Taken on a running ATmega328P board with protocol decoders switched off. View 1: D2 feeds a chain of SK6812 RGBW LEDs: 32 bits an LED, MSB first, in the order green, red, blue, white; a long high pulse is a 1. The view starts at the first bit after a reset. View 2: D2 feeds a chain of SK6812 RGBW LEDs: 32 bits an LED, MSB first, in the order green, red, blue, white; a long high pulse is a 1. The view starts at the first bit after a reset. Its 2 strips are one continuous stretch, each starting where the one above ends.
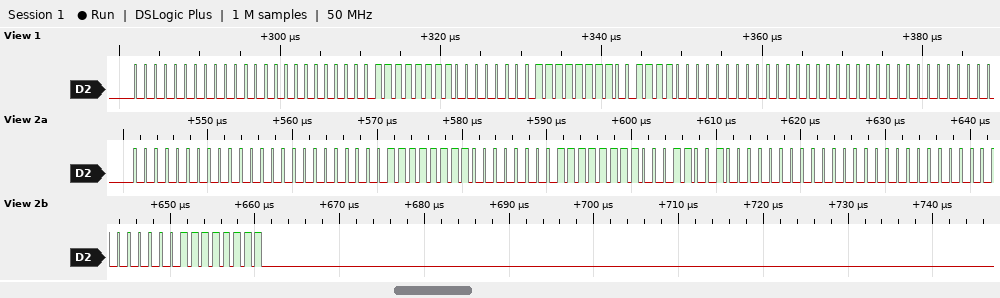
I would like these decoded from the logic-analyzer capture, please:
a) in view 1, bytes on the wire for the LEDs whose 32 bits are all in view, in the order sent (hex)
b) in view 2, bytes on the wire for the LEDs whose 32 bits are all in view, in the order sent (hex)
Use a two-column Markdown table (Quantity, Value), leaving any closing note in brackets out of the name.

| Quantity | Value |
|---|---|
| in view 1, bytes on the wire for the LEDs whose 32 bits are all in view, in the order sent | 00 00 00 FF 00 FF 3C 00 |
| in view 2, bytes on the wire for the LEDs whose 32 bits are all in view, in the order sent | 00 00 00 FF 00 FF 19 00 00 00 00 FF |
